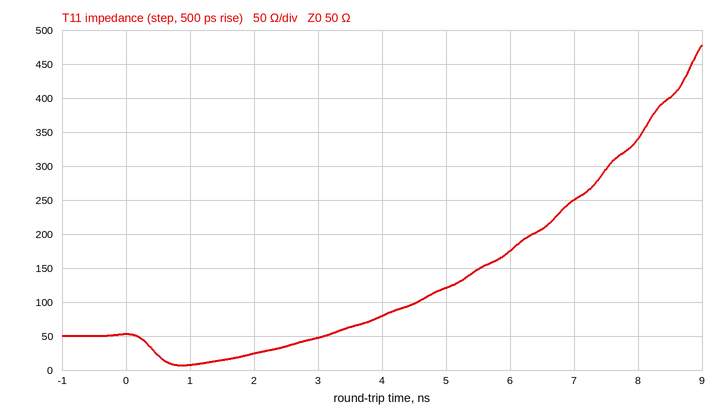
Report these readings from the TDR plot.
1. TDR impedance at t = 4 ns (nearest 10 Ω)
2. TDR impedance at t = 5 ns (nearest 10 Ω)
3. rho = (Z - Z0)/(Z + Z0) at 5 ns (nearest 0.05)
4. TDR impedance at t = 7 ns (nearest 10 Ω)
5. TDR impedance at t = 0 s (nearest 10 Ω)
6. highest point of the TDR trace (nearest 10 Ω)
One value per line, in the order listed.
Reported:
80 Ω
120 Ω
+0.40
250 Ω
50 Ω
480 Ω
